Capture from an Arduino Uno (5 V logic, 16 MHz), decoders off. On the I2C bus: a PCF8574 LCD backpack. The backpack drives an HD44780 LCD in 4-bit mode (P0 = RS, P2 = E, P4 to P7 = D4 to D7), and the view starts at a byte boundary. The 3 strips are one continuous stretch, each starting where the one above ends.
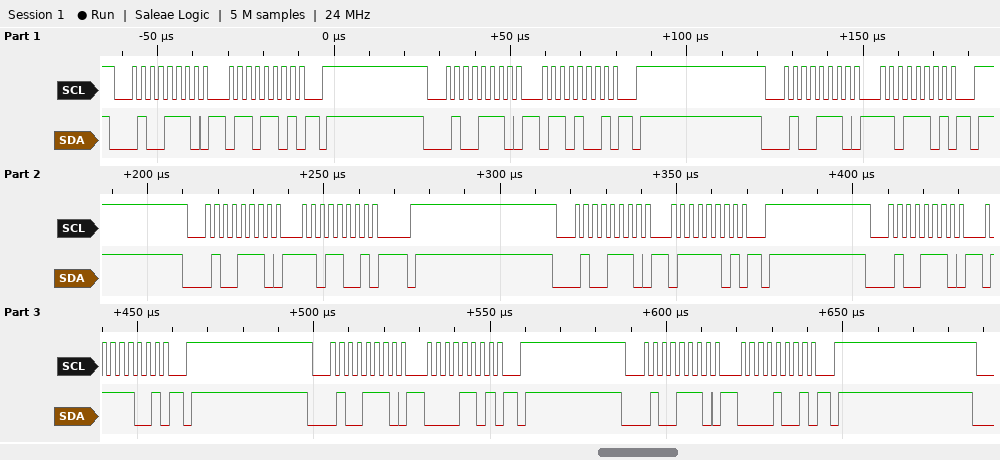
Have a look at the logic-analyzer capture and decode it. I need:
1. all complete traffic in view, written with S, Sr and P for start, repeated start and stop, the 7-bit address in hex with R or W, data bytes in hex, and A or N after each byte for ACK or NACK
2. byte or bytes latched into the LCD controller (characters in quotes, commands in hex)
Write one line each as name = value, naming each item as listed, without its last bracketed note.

all complete traffic in view, written with S, Sr and P for start, repeated start and stop, the 7-bit address in hex with R or W, data bytes in hex, and A or N after each byte for ACK or NACK = S 27W A 6D A P S 27W A 69 A P S 27W A DD A P S 27W A D9 A P S 27W A 7D A P S 27W A 79 A P S 27W A 0D A P S 27W A 09 A P
byte or bytes latched into the LCD controller = 'm' 'p'
